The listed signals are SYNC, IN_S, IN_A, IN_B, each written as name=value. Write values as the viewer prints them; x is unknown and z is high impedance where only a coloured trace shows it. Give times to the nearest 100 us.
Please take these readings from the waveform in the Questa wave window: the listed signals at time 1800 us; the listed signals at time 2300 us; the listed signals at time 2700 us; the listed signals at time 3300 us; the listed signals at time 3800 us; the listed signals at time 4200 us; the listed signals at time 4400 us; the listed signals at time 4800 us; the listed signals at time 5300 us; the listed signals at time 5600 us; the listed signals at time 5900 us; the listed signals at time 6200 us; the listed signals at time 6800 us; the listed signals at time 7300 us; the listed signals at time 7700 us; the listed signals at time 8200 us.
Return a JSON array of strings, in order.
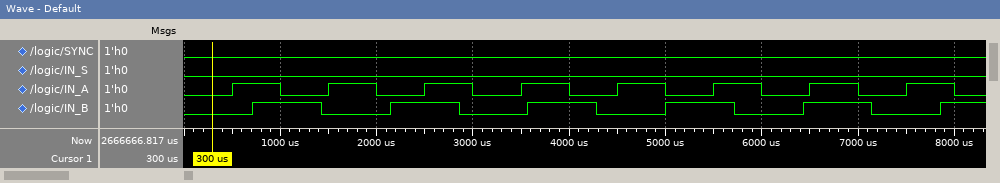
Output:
["SYNC=0, IN_S=0, IN_A=1, IN_B=0", "SYNC=0, IN_S=0, IN_A=0, IN_B=1", "SYNC=0, IN_S=0, IN_A=1, IN_B=1", "SYNC=0, IN_S=0, IN_A=0, IN_B=0", "SYNC=0, IN_S=0, IN_A=1, IN_B=1", "SYNC=0, IN_S=0, IN_A=0, IN_B=1", "SYNC=0, IN_S=0, IN_A=0, IN_B=0", "SYNC=0, IN_S=0, IN_A=1, IN_B=0", "SYNC=0, IN_S=0, IN_A=0, IN_B=1", "SYNC=0, IN_S=0, IN_A=1, IN_B=1", "SYNC=0, IN_S=0, IN_A=1, IN_B=0", "SYNC=0, IN_S=0, IN_A=0, IN_B=0", "SYNC=0, IN_S=0, IN_A=1, IN_B=1", "SYNC=0, IN_S=0, IN_A=0, IN_B=0", "SYNC=0, IN_S=0, IN_A=1, IN_B=0", "SYNC=0, IN_S=0, IN_A=0, IN_B=1"]
